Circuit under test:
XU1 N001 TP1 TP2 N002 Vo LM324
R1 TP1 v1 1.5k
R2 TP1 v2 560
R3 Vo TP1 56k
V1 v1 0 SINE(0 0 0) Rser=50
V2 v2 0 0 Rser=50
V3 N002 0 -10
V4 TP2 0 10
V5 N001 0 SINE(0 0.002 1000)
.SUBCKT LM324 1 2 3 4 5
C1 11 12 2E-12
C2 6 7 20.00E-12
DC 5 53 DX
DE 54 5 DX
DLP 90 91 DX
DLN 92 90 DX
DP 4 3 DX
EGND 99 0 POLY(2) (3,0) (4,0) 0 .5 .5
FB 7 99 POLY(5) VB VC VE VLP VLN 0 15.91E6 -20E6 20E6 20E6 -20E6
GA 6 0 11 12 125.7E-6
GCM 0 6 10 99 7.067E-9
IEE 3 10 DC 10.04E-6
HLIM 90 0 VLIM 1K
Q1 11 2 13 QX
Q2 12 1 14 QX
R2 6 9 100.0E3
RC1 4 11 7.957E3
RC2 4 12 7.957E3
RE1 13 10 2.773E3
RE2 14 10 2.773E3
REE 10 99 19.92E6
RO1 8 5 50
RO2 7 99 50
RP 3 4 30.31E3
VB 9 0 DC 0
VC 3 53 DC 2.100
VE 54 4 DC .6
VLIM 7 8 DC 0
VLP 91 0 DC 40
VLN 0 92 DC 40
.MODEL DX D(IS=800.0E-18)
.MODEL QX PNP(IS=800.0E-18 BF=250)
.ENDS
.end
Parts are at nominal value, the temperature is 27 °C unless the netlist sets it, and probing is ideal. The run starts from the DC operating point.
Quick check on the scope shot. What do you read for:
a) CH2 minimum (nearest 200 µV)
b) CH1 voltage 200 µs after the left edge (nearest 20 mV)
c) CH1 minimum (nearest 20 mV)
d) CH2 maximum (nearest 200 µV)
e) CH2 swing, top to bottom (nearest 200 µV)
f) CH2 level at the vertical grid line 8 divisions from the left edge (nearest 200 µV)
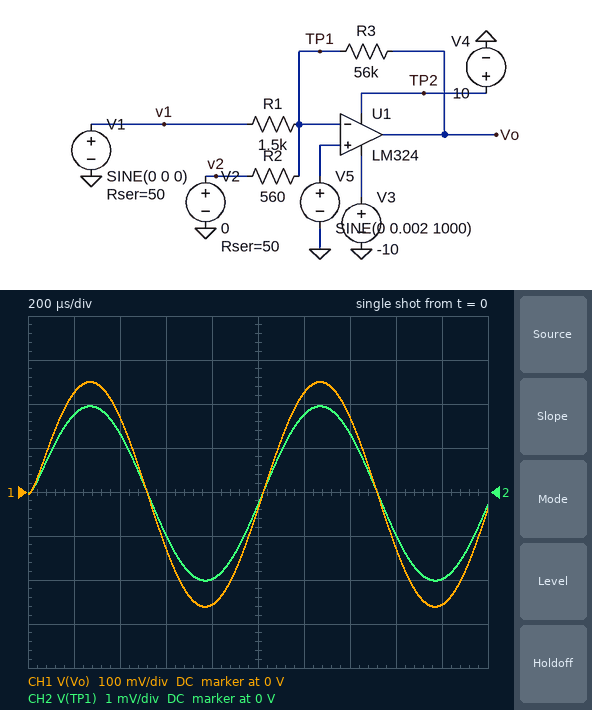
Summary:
-2.0 mV
220 mV
-260 mV
2.0 mV
4.0 mV
-1.0 mV
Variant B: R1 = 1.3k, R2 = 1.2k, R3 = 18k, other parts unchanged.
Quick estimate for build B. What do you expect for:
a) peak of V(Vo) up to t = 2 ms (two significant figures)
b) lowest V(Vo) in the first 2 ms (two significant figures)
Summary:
56 mV
-59 mV
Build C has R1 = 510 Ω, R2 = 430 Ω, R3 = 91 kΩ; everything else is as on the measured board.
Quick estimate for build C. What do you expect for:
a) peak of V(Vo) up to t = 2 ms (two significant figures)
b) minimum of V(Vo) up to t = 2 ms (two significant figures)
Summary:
650 mV
-680 mV
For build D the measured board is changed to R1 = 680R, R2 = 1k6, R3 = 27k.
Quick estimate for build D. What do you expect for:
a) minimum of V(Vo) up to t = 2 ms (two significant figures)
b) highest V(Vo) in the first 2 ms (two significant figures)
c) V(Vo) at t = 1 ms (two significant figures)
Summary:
-110 mV
110 mV
-8.3 mV
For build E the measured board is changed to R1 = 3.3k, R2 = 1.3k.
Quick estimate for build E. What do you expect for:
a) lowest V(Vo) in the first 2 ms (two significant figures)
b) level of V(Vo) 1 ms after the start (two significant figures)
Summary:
-120 mV
-10 mV
